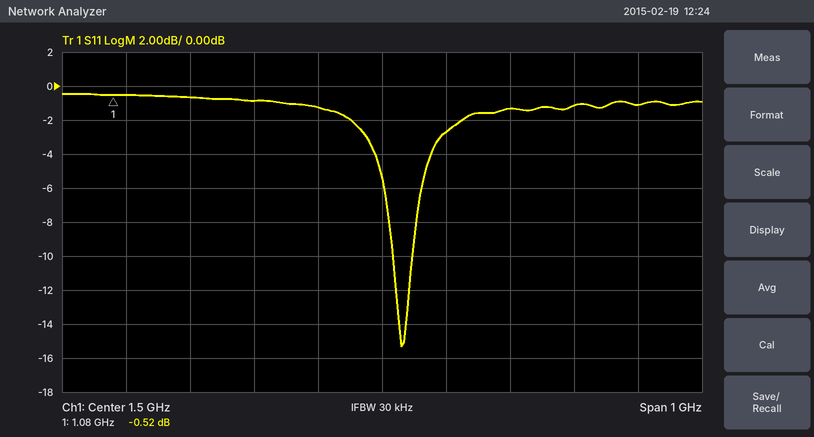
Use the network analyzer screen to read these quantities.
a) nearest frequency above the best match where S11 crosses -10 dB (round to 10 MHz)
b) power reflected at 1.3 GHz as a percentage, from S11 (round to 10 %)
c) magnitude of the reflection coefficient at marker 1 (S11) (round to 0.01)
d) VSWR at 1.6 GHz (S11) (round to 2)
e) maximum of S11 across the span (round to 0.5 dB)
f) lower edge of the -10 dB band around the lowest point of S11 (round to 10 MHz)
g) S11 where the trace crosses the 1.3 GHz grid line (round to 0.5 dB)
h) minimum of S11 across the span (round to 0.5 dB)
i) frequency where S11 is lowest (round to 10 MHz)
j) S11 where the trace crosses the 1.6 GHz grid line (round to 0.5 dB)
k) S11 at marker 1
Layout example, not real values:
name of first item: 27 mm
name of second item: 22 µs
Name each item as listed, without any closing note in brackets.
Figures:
nearest frequency above the best match where S11 crosses -10 dB: 1.55 GHz
power reflected at 1.3 GHz as a percentage, from S11: 80 %
magnitude of the reflection coefficient at marker 1 (S11): 0.94
VSWR at 1.6 GHz (S11): 6
maximum of S11 across the span: -0.5 dB
lower edge of the -10 dB band around the lowest point of S11: 1.52 GHz
S11 where the trace crosses the 1.3 GHz grid line: -1.0 dB
minimum of S11 across the span: -15.5 dB
frequency where S11 is lowest: 1.53 GHz
S11 where the trace crosses the 1.6 GHz grid line: -2.5 dB
S11 at marker 1: -0.52 dB
